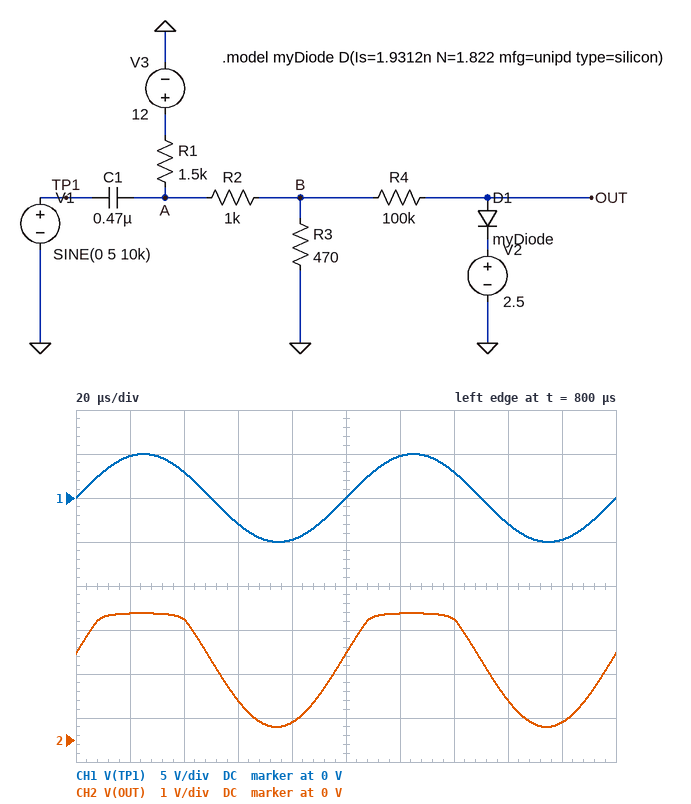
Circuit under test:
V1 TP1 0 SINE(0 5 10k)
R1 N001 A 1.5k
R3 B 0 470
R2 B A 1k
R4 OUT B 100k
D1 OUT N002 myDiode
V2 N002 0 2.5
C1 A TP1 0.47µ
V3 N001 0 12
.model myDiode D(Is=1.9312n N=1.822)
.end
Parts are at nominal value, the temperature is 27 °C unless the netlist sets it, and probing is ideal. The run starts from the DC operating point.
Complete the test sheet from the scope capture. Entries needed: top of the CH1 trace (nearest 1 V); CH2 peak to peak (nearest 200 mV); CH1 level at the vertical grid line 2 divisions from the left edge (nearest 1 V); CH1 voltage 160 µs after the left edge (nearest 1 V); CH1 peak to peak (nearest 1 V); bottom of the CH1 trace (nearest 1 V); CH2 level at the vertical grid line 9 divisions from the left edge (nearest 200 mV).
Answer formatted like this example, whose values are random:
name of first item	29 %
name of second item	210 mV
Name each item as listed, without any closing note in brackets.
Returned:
top of the CH1 trace	5 V
CH2 peak to peak	2.6 V
CH1 level at the vertical grid line 2 divisions from the left edge	3 V
CH1 voltage 160 µs after the left edge	-3 V
CH1 peak to peak	10 V
bottom of the CH1 trace	-5 V
CH2 level at the vertical grid line 9 divisions from the left edge	400 mV
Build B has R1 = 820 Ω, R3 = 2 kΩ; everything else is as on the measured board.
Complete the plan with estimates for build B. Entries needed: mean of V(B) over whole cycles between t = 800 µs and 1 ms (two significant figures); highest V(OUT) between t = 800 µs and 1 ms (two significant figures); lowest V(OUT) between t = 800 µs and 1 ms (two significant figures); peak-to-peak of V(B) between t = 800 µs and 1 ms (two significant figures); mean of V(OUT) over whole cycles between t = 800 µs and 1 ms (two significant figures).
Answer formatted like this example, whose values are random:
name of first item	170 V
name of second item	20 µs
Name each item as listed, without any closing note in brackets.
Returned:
mean of V(B) over whole cycles between t = 800 µs and 1 ms	6.2 V
highest V(OUT) between t = 800 µs and 1 ms	3.0 V
lowest V(OUT) between t = 800 µs and 1 ms	2.8 V
peak-to-peak of V(B) between t = 800 µs and 1 ms	6.6 V
mean of V(OUT) over whole cycles between t = 800 µs and 1 ms	2.9 V
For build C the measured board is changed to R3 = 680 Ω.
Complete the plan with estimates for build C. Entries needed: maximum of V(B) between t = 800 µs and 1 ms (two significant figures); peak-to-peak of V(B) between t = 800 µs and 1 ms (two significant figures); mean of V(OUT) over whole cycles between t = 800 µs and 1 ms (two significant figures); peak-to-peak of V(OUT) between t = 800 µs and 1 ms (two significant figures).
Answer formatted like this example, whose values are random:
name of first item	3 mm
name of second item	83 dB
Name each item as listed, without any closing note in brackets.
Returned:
maximum of V(B) between t = 800 µs and 1 ms	4.6 V
peak-to-peak of V(B) between t = 800 µs and 1 ms	4.0 V
mean of V(OUT) over whole cycles between t = 800 µs and 1 ms	2.1 V
peak-to-peak of V(OUT) between t = 800 µs and 1 ms	2.4 V
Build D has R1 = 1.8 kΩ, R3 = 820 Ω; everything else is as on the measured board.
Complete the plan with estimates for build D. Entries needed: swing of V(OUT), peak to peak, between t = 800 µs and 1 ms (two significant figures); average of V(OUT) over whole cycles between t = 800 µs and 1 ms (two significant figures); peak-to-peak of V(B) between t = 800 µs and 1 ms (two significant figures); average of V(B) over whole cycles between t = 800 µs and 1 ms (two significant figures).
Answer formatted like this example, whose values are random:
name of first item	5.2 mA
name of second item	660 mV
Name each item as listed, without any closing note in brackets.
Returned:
swing of V(OUT), peak to peak, between t = 800 µs and 1 ms	2.5 V
average of V(OUT) over whole cycles between t = 800 µs and 1 ms	2.1 V
peak-to-peak of V(B) between t = 800 µs and 1 ms	4.5 V
average of V(B) over whole cycles between t = 800 µs and 1 ms	2.7 V
